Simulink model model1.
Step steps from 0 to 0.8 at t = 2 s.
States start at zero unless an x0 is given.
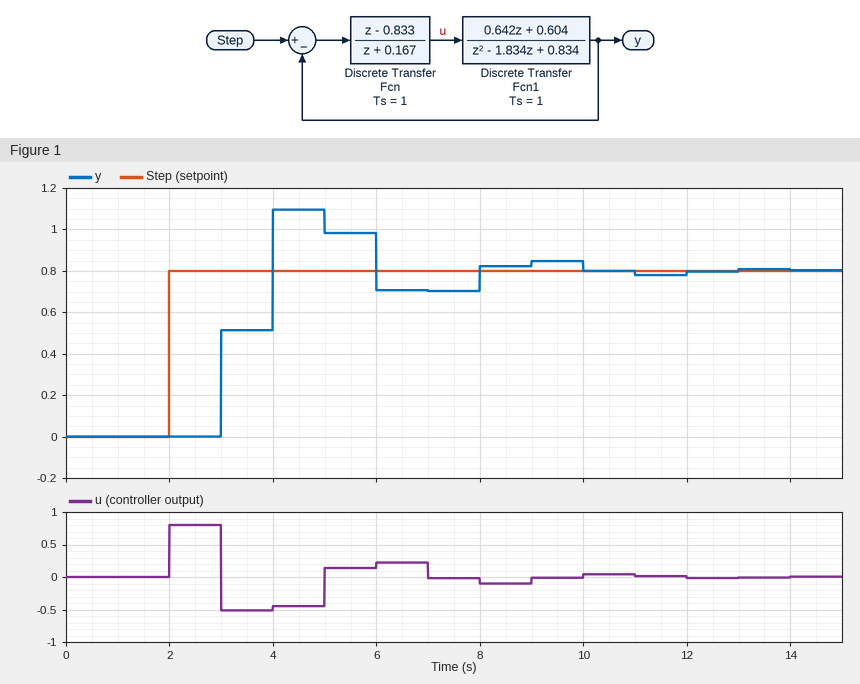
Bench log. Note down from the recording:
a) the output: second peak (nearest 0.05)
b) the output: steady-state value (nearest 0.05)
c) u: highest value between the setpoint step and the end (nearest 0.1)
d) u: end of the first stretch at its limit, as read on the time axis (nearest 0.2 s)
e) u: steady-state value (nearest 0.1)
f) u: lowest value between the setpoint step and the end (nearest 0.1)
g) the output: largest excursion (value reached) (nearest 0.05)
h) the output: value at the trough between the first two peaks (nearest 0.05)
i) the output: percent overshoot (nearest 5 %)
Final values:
0.85
0.80
0.8
3.0 s
0.0
-0.5
1.10
0.70
35 %
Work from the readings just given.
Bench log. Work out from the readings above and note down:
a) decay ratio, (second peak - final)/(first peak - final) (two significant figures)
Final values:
0.17
